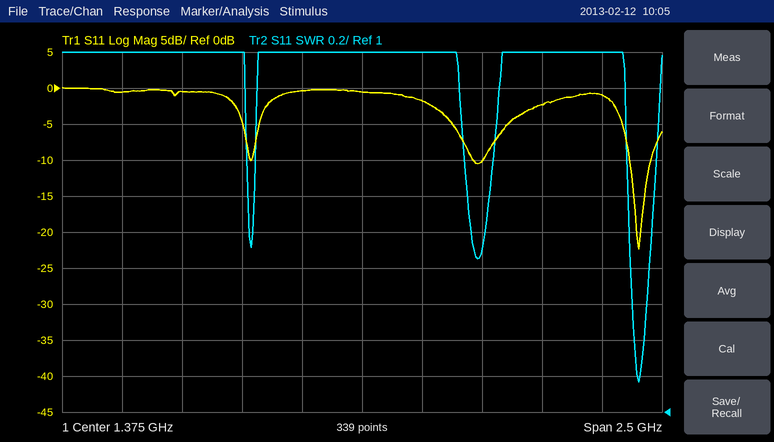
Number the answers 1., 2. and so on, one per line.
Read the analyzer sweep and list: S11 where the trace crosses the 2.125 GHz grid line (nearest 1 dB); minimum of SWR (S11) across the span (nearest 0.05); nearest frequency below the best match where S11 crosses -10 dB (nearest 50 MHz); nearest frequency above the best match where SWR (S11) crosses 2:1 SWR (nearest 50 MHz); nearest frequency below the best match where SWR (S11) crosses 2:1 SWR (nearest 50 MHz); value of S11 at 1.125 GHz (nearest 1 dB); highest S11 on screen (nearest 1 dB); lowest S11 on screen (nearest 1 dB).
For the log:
1. -2 dB
2. 1.15
3. 2.50 GHz
4. 2.60 GHz
5. 2.50 GHz
6. 0 dB
7. 0 dB
8. -22 dB
